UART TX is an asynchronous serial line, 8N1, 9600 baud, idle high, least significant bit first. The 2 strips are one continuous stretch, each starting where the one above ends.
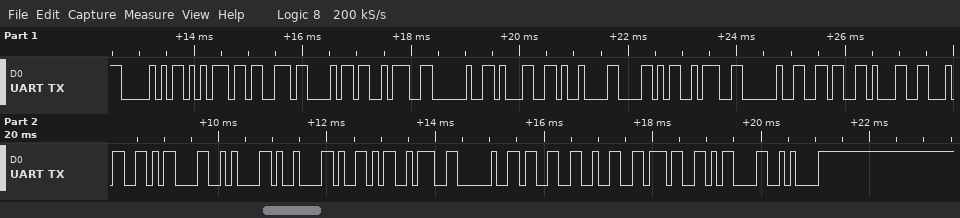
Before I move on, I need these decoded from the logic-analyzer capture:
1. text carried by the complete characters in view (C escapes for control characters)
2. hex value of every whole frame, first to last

"Push: 1\tX: 614\r\n\tY: 327\r\n"
50 75 73 68 3A 20 31 09 58 3A 20 36 31 34 0D 0A 09 59 3A 20 33 32 37 0D 0A
